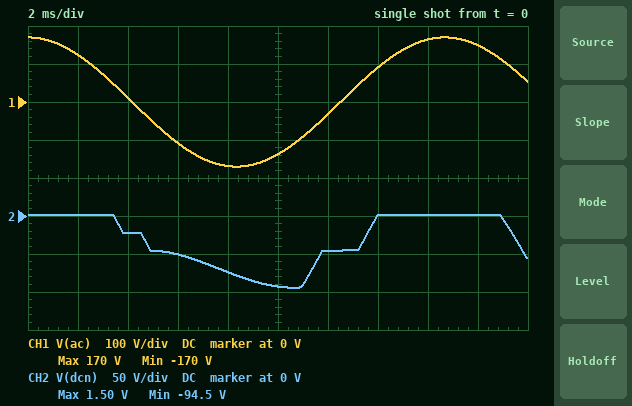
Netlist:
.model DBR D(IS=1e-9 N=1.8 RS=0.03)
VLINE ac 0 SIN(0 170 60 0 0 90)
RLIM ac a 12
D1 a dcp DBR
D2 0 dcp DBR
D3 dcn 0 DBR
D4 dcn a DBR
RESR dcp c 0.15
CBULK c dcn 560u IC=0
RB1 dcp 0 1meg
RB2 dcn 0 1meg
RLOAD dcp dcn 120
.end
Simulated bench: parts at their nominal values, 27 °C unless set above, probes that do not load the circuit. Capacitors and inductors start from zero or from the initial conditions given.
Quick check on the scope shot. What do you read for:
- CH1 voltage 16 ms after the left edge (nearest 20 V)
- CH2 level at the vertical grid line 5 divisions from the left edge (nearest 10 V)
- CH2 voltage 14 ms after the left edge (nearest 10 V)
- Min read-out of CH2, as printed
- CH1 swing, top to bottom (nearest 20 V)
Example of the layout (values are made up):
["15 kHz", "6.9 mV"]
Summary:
["160 V", "-90 V", "0 V", "-94.5 V", "340 V"]
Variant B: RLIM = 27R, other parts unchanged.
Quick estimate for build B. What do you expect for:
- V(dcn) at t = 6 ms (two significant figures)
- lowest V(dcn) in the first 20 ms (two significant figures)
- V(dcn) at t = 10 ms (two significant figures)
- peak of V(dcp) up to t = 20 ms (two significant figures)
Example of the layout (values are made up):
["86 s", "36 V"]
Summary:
["-29 V", "-58 V", "-55 V", "77 V"]
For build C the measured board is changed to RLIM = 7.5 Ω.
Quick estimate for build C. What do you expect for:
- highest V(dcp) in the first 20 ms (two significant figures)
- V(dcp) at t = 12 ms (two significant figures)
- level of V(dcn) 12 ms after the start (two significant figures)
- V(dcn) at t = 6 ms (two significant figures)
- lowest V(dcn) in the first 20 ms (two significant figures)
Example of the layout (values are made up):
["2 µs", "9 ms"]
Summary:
["130 V", "56 V", "-56 V", "-66 V", "-120 V"]
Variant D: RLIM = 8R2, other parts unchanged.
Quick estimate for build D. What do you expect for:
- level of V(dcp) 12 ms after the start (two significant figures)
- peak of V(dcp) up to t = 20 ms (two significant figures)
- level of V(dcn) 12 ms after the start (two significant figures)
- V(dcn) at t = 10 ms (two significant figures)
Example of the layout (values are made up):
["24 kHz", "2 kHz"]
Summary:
["54 V", "130 V", "-54 V", "-110 V"]
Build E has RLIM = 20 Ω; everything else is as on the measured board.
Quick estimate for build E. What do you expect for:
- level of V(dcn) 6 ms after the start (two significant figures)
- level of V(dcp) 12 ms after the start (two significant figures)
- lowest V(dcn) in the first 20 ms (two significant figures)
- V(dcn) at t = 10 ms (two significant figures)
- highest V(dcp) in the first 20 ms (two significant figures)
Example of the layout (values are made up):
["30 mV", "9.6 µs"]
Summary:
["-36 V", "34 V", "-71 V", "-68 V", "91 V"]
